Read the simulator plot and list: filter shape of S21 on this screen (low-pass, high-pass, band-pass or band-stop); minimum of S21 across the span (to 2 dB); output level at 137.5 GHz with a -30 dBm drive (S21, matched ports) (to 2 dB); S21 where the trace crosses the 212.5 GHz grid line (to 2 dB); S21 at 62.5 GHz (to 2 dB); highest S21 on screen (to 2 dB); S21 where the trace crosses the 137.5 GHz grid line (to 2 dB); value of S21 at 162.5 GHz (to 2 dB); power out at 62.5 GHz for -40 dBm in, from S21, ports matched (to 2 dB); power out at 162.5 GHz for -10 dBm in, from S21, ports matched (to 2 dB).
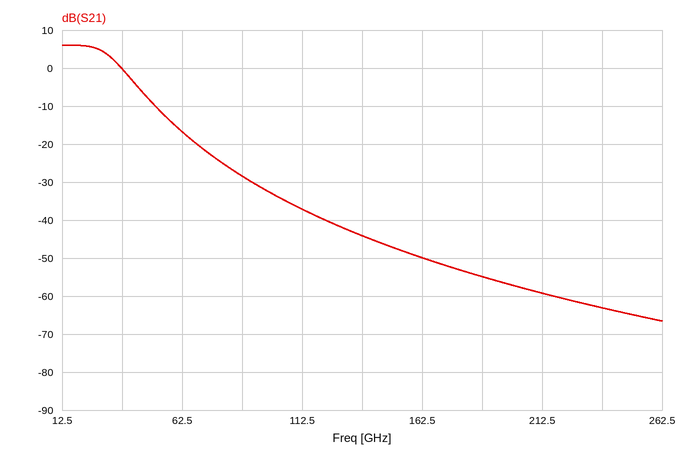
low-pass
-66 dB
-74 dBm
-60 dB
-16 dB
6 dB
-44 dB
-50 dB
-56 dBm
-60 dBm
